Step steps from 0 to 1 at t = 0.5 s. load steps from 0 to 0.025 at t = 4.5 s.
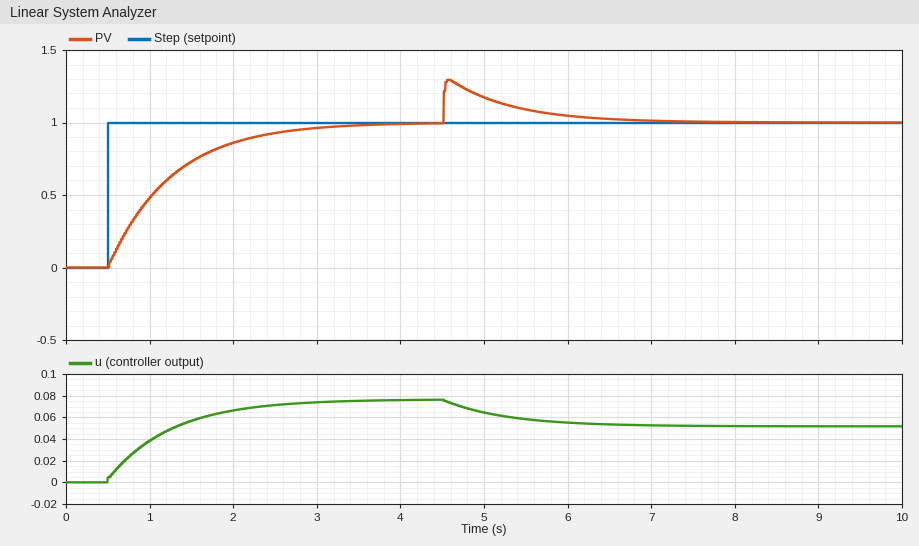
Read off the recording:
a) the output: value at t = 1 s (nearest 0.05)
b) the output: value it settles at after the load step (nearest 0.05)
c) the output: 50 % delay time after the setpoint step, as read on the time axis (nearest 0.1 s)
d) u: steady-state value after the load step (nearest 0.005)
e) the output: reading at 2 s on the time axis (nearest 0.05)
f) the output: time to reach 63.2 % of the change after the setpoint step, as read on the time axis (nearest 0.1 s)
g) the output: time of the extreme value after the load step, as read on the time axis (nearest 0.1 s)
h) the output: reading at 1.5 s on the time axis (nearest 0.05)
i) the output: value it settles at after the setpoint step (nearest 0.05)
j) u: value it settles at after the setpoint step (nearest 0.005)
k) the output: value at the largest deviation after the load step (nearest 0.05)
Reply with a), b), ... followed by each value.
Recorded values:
a) 0.50
b) 1.00
c) 1.0 s
d) 0.050
e) 0.85
f) 1.3 s
g) 4.6 s
h) 0.75
i) 1.00
j) 0.075
k) 1.30
